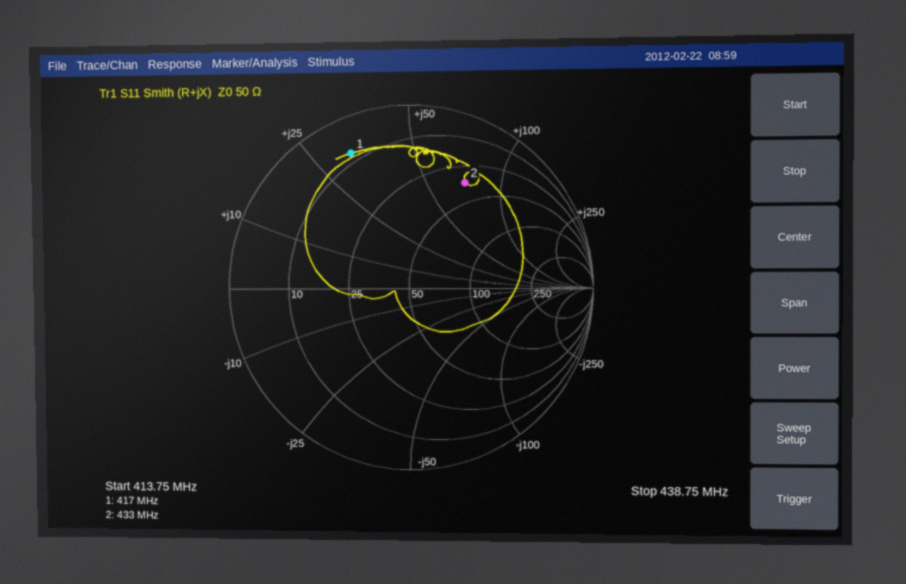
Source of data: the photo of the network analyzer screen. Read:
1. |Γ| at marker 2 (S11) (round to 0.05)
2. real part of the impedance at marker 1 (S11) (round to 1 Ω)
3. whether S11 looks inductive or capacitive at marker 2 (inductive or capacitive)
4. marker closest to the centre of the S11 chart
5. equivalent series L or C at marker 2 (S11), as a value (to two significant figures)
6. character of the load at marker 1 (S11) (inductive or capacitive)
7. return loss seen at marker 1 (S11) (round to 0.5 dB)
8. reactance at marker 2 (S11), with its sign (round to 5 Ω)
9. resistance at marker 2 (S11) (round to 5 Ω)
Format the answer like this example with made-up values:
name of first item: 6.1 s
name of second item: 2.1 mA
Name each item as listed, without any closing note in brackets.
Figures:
|Γ| at marker 2 (S11): 0.65
real part of the impedance at marker 1 (S11): 8 Ω
whether S11 looks inductive or capacitive at marker 2: inductive
marker closest to the centre of the S11 chart: marker 2
equivalent series L or C at marker 2 (S11), as a value: 26 nH
character of the load at marker 1 (S11): inductive
return loss seen at marker 1 (S11): 2.0 dB
reactance at marker 2 (S11), with its sign: +70 Ω
resistance at marker 2 (S11): 35 Ω
